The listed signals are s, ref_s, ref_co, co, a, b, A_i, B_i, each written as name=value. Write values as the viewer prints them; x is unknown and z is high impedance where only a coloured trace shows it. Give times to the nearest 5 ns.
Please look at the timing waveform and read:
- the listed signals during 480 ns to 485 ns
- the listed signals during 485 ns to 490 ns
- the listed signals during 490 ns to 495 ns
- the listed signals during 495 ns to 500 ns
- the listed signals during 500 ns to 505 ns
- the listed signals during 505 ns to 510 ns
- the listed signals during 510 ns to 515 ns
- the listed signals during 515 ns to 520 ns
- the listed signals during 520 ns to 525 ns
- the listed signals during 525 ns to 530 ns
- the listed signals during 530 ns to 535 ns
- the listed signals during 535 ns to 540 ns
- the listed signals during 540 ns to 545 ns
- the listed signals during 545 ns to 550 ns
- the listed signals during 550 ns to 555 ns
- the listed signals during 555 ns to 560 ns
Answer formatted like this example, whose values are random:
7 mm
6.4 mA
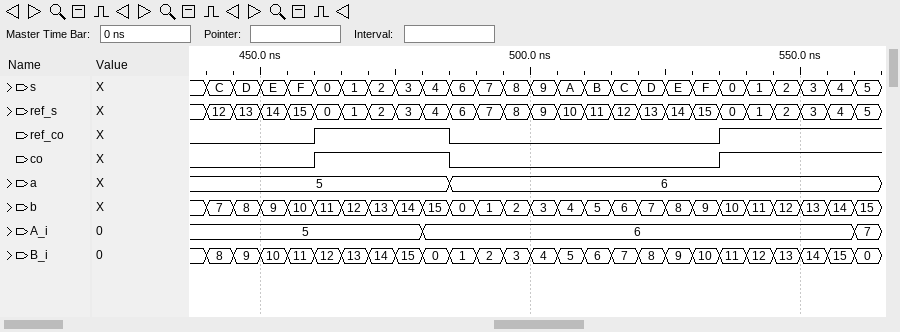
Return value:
s=4, ref_s=4, ref_co=1, co=1, a=5, b=15, A_i=6, B_i=0
s=6, ref_s=6, ref_co=0, co=0, a=6, b=0, A_i=6, B_i=1
s=7, ref_s=7, ref_co=0, co=0, a=6, b=1, A_i=6, B_i=2
s=8, ref_s=8, ref_co=0, co=0, a=6, b=2, A_i=6, B_i=3
s=9, ref_s=9, ref_co=0, co=0, a=6, b=3, A_i=6, B_i=4
s=A, ref_s=10, ref_co=0, co=0, a=6, b=4, A_i=6, B_i=5
s=B, ref_s=11, ref_co=0, co=0, a=6, b=5, A_i=6, B_i=6
s=C, ref_s=12, ref_co=0, co=0, a=6, b=6, A_i=6, B_i=7
s=D, ref_s=13, ref_co=0, co=0, a=6, b=7, A_i=6, B_i=8
s=E, ref_s=14, ref_co=0, co=0, a=6, b=8, A_i=6, B_i=9
s=F, ref_s=15, ref_co=0, co=0, a=6, b=9, A_i=6, B_i=10
s=0, ref_s=0, ref_co=1, co=1, a=6, b=10, A_i=6, B_i=11
s=1, ref_s=1, ref_co=1, co=1, a=6, b=11, A_i=6, B_i=12
s=2, ref_s=2, ref_co=1, co=1, a=6, b=12, A_i=6, B_i=13
s=3, ref_s=3, ref_co=1, co=1, a=6, b=13, A_i=6, B_i=14
s=4, ref_s=4, ref_co=1, co=1, a=6, b=14, A_i=6, B_i=15
